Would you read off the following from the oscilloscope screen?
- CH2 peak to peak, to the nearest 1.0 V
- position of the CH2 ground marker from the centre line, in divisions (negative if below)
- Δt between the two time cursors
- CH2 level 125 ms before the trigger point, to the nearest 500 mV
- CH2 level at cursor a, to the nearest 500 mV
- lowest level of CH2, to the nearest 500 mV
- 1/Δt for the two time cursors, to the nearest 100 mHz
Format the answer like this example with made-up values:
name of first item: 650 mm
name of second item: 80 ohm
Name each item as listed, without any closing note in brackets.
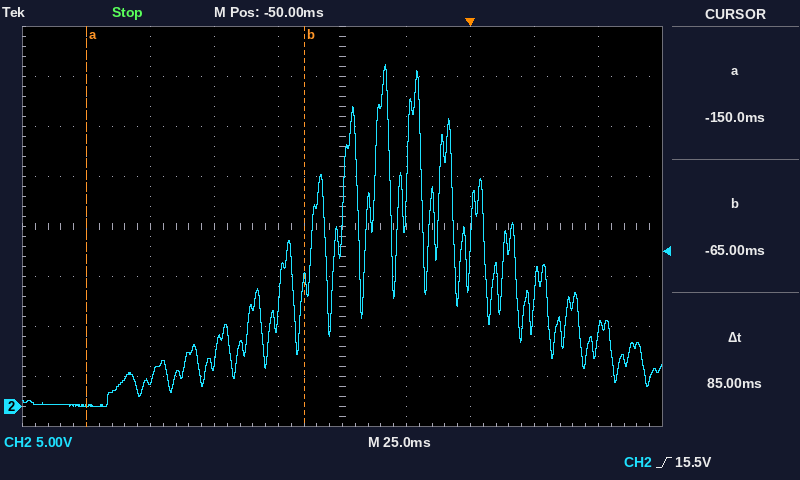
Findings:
CH2 peak to peak, to the nearest 1.0 V: 34.0 V
position of the CH2 ground marker from the centre line, in divisions: -3.6 div
Δt between the two time cursors: 85 ms
CH2 level 125 ms before the trigger point, to the nearest 500 mV: 2.5 V
CH2 level at cursor a, to the nearest 500 mV: 0.0 V
lowest level of CH2, to the nearest 500 mV: 0.0 V
1/Δt for the two time cursors, to the nearest 100 mHz: 11.8 Hz
